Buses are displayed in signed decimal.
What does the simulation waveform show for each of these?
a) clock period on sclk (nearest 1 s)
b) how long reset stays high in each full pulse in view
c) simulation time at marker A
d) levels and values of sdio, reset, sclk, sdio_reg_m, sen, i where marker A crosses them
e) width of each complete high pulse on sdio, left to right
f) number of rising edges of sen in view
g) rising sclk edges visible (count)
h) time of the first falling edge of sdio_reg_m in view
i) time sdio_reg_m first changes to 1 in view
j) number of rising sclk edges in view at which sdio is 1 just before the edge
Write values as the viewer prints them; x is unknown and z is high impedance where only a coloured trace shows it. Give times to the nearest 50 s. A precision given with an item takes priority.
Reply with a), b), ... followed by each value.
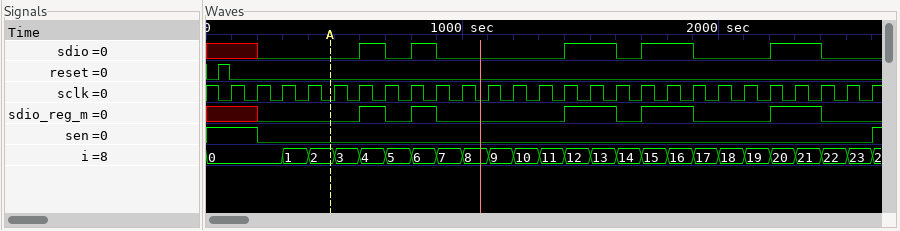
a) 100 s
b) 50 s
c) 500 s
d) sdio=0, reset=0, sclk=0, sdio_reg_m=0, sen=0, i=2
e) 100 s, 100 s, 200 s, 200 s, 200 s
f) 1
g) 26
h) 700 s
i) 600 s
j) 8
